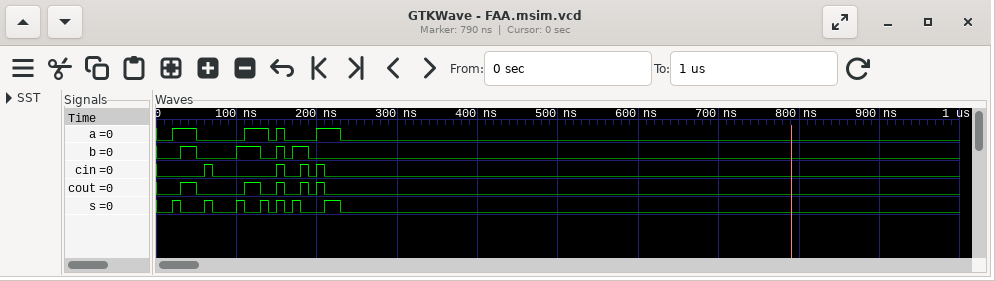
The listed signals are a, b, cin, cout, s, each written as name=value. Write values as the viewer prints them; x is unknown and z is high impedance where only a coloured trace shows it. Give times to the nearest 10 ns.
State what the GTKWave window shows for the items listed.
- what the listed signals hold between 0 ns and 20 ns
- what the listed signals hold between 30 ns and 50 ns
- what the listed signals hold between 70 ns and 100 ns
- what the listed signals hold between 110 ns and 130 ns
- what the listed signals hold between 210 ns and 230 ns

a=0, b=0, cin=0, cout=0, s=0
a=1, b=1, cin=0, cout=1, s=0
a=0, b=0, cin=0, cout=0, s=0
a=1, b=1, cin=0, cout=1, s=0
a=1, b=0, cin=0, cout=0, s=1
